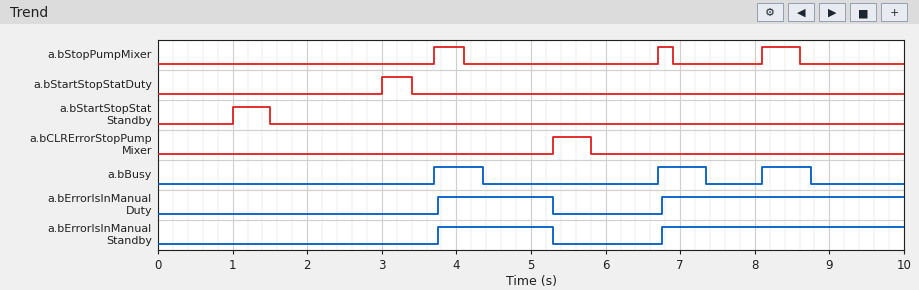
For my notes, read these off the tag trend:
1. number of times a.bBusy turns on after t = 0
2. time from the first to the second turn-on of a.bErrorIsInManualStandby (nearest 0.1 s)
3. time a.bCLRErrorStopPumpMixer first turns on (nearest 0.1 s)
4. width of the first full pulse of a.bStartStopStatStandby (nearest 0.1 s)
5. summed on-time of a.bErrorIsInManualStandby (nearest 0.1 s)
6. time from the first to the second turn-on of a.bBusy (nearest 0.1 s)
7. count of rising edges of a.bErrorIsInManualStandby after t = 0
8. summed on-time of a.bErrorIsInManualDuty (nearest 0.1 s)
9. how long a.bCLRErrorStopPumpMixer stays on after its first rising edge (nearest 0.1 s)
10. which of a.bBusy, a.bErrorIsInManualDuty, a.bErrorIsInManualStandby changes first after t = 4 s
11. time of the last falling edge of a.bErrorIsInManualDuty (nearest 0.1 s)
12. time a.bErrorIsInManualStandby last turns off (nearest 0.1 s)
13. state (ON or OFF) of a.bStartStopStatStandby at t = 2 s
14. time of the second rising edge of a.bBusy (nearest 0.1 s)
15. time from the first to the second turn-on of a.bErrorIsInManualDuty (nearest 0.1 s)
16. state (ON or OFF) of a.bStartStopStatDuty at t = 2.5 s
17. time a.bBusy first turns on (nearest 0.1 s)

3
3.0 s
5.3 s
0.5 s
4.8 s
3.0 s
2
4.8 s
0.5 s
a.bBusy
5.3 s
5.3 s
OFF
6.7 s
3.0 s
OFF
3.7 s
